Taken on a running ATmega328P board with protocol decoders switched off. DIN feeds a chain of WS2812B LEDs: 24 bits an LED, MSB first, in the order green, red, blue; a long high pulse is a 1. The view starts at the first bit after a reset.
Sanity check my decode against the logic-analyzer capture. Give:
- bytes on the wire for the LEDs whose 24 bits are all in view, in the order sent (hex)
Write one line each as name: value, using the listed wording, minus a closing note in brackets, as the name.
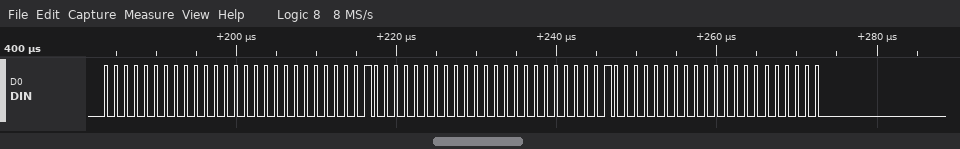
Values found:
bytes on the wire for the LEDs whose 24 bits are all in view, in the order sent: 00 00 00 20 00 00 20 00 00
